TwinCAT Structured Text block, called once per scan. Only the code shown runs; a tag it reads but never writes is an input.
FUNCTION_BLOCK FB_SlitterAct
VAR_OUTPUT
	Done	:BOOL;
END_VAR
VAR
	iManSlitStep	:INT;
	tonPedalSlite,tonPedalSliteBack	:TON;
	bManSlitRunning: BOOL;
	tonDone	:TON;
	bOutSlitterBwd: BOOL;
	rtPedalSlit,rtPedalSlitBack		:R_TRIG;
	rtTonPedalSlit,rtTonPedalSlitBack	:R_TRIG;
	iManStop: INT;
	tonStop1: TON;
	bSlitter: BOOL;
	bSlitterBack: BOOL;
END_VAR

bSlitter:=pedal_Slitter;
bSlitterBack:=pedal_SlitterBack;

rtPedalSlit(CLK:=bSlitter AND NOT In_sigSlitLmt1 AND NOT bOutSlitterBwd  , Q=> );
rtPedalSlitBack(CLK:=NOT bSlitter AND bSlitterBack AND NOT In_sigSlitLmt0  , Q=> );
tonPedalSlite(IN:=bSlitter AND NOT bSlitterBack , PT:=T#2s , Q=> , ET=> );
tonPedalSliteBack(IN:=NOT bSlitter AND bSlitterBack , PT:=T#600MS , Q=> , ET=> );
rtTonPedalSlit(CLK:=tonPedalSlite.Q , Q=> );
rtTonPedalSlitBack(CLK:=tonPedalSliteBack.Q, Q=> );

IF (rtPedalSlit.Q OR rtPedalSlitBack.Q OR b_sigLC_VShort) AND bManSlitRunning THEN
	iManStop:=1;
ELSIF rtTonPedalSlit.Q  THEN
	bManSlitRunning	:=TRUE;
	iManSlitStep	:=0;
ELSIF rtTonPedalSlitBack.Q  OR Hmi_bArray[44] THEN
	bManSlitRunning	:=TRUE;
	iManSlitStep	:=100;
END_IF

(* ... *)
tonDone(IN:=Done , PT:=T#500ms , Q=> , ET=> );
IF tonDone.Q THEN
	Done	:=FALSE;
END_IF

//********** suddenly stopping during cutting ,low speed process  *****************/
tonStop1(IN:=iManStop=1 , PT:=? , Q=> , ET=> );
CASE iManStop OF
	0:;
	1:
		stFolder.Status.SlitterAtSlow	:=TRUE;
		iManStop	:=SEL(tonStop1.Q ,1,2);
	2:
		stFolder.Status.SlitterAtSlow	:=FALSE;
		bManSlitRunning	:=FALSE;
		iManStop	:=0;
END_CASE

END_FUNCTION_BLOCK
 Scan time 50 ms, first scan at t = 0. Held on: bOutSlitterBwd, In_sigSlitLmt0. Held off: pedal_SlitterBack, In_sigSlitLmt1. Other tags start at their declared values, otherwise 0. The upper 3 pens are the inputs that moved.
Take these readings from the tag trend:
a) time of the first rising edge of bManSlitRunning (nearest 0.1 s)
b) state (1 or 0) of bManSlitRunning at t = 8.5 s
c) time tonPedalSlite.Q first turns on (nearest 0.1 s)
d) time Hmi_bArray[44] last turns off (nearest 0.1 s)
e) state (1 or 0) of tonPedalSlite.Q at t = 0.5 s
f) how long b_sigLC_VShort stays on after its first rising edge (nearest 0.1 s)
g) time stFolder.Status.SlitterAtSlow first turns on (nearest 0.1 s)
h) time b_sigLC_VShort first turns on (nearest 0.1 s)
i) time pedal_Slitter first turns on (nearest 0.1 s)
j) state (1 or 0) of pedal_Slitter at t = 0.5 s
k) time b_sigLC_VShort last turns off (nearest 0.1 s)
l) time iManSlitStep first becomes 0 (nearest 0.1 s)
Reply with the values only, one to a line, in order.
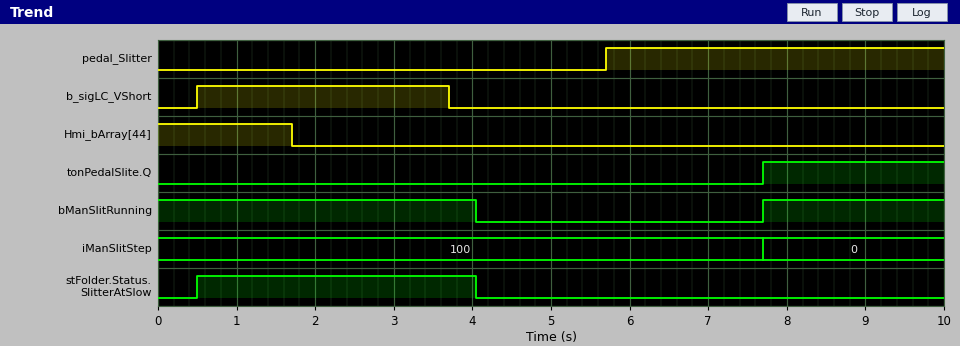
7.7 s
1
7.7 s
1.7 s
0
3.2 s
0.5 s
0.5 s
5.7 s
0
3.7 s
7.7 s
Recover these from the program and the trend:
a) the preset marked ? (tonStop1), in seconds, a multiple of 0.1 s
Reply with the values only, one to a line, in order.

3.5 s
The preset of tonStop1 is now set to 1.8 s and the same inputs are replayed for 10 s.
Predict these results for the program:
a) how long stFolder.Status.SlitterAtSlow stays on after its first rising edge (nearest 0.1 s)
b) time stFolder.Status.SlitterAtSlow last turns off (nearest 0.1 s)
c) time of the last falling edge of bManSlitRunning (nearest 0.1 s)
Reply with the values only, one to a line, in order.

3.2 s
3.7 s
3.7 s
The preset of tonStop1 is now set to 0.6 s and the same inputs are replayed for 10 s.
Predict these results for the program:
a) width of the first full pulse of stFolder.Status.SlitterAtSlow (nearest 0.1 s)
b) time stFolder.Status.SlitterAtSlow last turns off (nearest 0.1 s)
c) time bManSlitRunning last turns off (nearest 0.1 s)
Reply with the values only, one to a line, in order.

3.2 s
3.7 s
3.7 s
